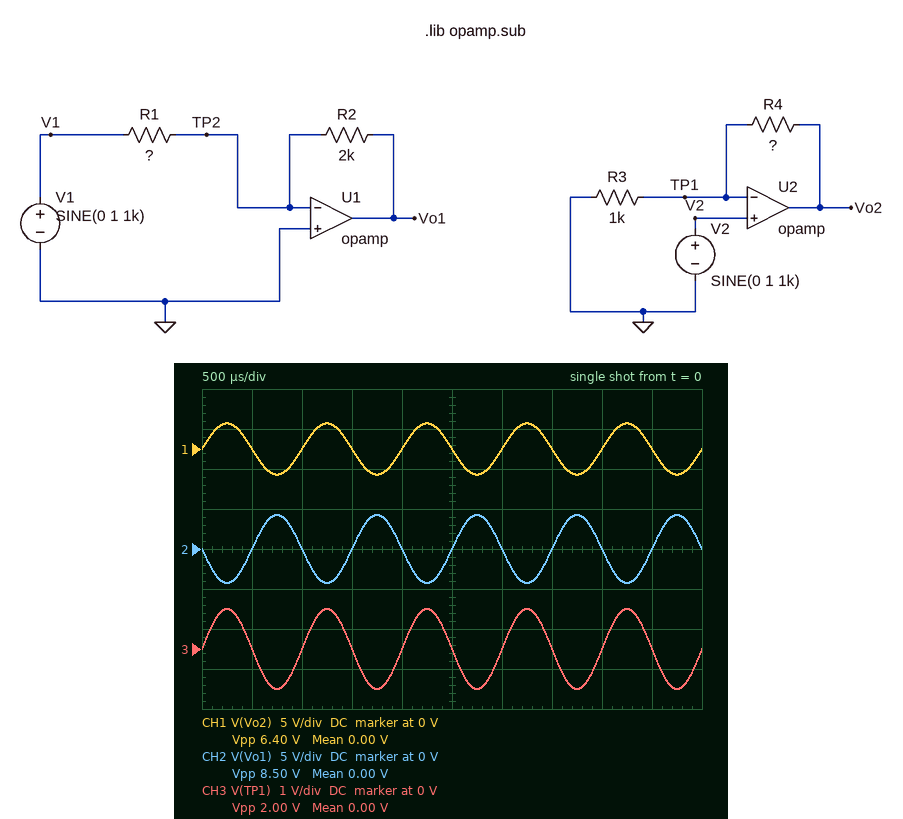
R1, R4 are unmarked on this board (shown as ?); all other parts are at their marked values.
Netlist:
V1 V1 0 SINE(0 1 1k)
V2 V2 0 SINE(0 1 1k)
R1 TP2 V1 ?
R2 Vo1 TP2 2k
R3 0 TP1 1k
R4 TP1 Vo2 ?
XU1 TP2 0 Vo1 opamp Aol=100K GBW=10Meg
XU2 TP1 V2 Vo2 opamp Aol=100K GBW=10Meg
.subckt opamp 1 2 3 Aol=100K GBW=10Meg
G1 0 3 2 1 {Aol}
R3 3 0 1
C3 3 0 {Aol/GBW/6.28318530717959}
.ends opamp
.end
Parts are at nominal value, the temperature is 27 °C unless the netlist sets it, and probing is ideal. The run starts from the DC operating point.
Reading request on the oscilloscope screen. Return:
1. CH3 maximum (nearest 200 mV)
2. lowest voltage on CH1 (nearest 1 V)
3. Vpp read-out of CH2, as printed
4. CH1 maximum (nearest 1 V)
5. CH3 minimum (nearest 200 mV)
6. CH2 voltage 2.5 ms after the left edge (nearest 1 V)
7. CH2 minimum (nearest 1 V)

1.0 V
-3 V
8.50 V
3 V
-1.0 V
0 V
-4 V
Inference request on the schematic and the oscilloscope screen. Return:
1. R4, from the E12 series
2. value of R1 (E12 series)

2.2 kΩ
470 Ω
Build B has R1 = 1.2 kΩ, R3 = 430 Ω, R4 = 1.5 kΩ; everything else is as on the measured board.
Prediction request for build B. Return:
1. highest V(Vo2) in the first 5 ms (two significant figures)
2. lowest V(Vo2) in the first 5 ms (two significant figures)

4.5 V
-4.5 V
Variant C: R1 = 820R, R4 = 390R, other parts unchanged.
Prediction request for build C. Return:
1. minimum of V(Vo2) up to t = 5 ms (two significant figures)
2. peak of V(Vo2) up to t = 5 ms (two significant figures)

-1.4 V
1.4 V
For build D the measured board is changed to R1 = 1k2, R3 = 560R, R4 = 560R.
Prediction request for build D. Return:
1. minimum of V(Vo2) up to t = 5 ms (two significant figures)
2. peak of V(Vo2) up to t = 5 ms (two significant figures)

-2.0 V
2.0 V
